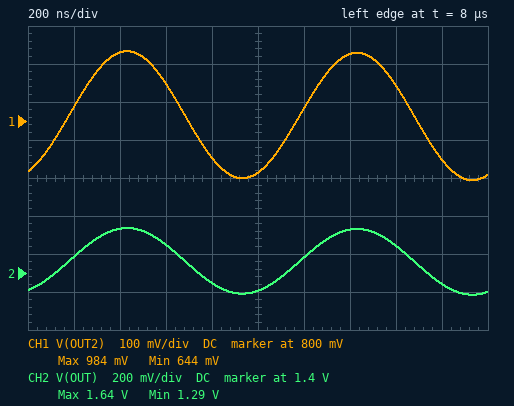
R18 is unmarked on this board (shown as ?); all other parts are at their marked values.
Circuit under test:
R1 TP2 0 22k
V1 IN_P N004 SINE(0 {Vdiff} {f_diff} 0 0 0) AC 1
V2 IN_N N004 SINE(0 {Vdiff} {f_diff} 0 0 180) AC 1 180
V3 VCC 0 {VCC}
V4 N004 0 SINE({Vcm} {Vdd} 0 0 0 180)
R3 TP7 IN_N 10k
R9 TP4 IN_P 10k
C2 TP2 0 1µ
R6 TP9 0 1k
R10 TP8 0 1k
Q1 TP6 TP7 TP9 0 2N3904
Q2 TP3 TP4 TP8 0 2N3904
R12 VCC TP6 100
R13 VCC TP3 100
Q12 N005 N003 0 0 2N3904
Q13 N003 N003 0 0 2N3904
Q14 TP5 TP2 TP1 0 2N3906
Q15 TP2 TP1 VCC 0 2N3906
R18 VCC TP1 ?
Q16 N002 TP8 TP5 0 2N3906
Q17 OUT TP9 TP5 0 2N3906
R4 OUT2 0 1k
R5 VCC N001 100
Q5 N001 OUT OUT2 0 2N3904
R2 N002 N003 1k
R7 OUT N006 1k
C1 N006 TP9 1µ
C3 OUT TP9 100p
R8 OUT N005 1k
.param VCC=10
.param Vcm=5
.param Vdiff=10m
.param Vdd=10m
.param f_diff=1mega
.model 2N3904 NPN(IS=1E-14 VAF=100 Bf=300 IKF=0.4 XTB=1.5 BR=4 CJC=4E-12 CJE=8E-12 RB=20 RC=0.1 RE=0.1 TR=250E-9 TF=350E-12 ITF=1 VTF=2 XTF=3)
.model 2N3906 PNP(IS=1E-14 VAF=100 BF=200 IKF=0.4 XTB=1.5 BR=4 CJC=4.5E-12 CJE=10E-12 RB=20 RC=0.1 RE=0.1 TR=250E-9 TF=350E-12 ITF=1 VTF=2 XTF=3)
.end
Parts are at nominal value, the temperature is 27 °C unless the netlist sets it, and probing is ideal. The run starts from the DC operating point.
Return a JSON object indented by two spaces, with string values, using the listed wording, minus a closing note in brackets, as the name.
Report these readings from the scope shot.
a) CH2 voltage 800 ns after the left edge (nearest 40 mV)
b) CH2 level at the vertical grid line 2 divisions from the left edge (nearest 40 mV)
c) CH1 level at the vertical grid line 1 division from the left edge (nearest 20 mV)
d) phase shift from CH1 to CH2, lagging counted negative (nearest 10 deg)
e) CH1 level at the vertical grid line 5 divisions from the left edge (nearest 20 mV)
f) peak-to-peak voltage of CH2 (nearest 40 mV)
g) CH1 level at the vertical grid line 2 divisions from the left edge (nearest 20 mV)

{
  "CH2 voltage 800 ns after the left edge": "1.36 V",
  "CH2 level at the vertical grid line 2 divisions from the left edge": "1.64 V",
  "CH1 level at the vertical grid line 1 division from the left edge": "840 mV",
  "phase shift from CH1 to CH2, lagging counted negative": "0 deg",
  "CH1 level at the vertical grid line 5 divisions from the left edge": "660 mV",
  "peak-to-peak voltage of CH2": "360 mV",
  "CH1 level at the vertical grid line 2 divisions from the left edge": "980 mV"
}
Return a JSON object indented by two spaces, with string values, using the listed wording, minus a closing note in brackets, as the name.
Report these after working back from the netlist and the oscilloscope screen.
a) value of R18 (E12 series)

{
  "value of R18": "470 Ω"
}
